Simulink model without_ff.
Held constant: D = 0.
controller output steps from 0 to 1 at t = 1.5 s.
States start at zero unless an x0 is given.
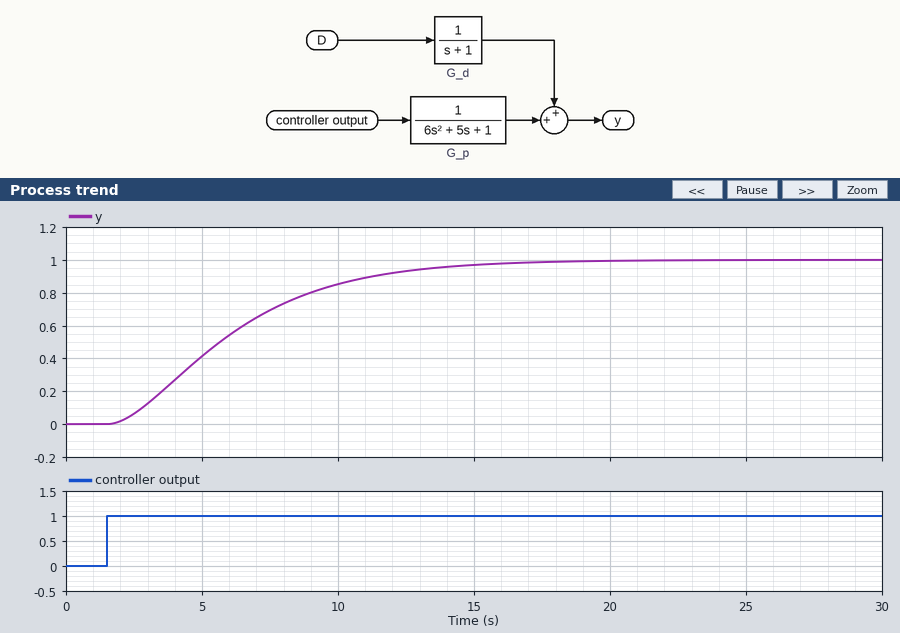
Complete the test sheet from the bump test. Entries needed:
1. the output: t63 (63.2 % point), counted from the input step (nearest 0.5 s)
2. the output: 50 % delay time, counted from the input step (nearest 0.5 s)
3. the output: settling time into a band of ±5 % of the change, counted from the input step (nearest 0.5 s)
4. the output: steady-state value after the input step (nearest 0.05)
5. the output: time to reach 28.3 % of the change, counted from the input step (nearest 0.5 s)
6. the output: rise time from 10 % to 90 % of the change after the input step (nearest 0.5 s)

5.5 s
4.0 s
12.0 s
1.00
2.5 s
8.5 s
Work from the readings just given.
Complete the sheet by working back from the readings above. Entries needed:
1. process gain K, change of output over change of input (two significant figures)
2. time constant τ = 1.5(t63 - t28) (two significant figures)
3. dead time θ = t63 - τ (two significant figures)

1.0
4.5 s
1.0 s
